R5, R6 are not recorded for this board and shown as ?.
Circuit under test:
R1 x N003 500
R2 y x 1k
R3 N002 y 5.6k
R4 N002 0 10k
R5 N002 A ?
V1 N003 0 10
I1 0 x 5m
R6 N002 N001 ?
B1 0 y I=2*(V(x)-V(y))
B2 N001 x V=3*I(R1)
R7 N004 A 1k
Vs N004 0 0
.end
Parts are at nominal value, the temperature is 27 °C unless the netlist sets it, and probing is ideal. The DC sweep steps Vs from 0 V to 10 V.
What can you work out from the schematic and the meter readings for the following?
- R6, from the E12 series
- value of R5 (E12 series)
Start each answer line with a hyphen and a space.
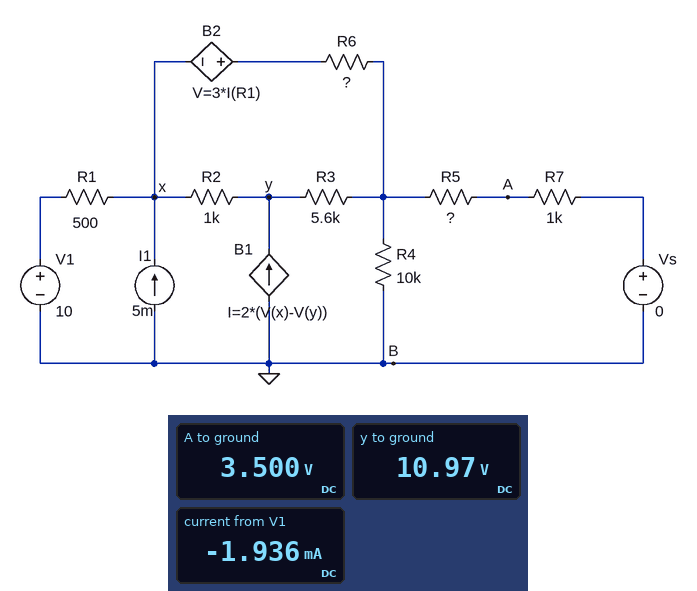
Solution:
- 1.8 kΩ
- 560 Ω
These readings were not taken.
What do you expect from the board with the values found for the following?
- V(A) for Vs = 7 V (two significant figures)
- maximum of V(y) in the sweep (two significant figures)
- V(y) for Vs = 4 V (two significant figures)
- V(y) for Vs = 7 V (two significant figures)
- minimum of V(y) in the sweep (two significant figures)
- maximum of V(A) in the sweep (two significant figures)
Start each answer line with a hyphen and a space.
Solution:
- 8.2 V
- 12 V
- 11 V
- 12 V
- 11 V
- 10 V
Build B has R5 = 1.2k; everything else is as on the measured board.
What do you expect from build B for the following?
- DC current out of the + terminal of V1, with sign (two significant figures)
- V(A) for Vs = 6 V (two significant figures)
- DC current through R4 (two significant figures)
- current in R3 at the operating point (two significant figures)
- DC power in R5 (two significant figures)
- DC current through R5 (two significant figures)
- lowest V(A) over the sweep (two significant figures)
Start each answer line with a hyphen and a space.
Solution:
- -2.3 mA
- 7.3 V
- 640 µA
- 860 µA
- 10 mW
- 2.9 mA
- 2.9 V
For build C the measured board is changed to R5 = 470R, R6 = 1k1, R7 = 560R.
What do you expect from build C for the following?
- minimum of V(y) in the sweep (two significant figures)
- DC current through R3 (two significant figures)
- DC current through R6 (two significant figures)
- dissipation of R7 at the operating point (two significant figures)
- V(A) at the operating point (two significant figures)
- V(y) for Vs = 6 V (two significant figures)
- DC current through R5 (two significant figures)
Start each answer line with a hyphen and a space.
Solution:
- 10 V
- 900 µA
- 4.6 mA
- 14 mW
- 2.8 V
- 11 V
- 5.0 mA
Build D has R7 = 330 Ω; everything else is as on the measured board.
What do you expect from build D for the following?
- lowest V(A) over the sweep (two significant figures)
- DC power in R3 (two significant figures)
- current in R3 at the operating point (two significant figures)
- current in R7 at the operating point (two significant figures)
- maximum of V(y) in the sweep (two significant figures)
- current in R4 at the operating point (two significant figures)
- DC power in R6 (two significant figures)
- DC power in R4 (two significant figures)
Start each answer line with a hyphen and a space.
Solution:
- 1.5 V
- 7.9 mW
- 1.2 mA
- 4.5 mA
- 12 V
- 400 µA
- 25 mW
- 1.6 mW
